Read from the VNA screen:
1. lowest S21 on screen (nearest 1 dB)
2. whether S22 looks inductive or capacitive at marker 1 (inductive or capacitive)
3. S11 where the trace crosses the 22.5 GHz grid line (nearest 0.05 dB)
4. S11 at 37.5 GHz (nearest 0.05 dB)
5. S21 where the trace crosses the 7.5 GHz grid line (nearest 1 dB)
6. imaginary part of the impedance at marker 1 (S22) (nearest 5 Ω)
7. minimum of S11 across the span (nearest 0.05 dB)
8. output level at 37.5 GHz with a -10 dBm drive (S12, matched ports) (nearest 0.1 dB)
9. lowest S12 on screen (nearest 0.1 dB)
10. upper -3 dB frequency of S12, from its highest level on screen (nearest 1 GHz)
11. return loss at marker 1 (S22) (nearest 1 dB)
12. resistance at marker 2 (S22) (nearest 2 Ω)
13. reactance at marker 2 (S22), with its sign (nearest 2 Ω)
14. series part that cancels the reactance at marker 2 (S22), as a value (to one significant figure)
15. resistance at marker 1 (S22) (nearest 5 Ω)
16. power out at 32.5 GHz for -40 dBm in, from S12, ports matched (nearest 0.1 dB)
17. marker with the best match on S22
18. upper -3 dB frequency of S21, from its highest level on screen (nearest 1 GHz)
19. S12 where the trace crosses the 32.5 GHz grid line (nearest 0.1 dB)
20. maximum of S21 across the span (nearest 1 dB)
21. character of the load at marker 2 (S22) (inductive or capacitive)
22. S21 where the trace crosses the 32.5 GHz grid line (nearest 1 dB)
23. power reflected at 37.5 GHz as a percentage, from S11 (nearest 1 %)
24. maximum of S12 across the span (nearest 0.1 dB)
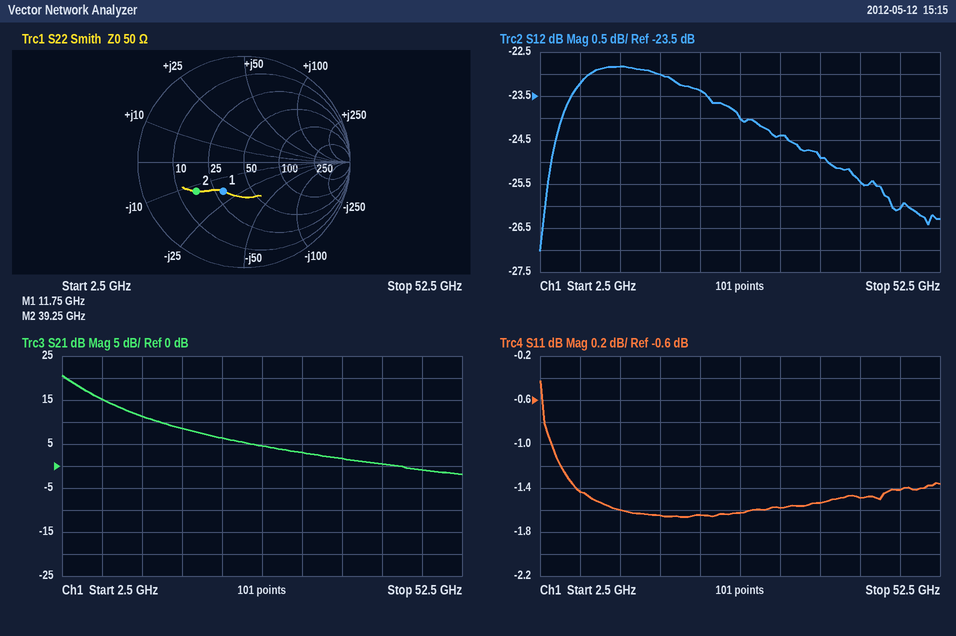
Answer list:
-2 dB
capacitive
-1.65 dB
-1.55 dB
15 dB
-20 Ω
-1.65 dB
-34.9 dBm
-27.0 dB
46 GHz
9 dB
16 Ω
-12 Ω
50 pH
30 Ω
-64.4 dBm
marker 1
5 GHz
-24.4 dB
21 dB
capacitive
3 dB
70 %
-22.8 dB
